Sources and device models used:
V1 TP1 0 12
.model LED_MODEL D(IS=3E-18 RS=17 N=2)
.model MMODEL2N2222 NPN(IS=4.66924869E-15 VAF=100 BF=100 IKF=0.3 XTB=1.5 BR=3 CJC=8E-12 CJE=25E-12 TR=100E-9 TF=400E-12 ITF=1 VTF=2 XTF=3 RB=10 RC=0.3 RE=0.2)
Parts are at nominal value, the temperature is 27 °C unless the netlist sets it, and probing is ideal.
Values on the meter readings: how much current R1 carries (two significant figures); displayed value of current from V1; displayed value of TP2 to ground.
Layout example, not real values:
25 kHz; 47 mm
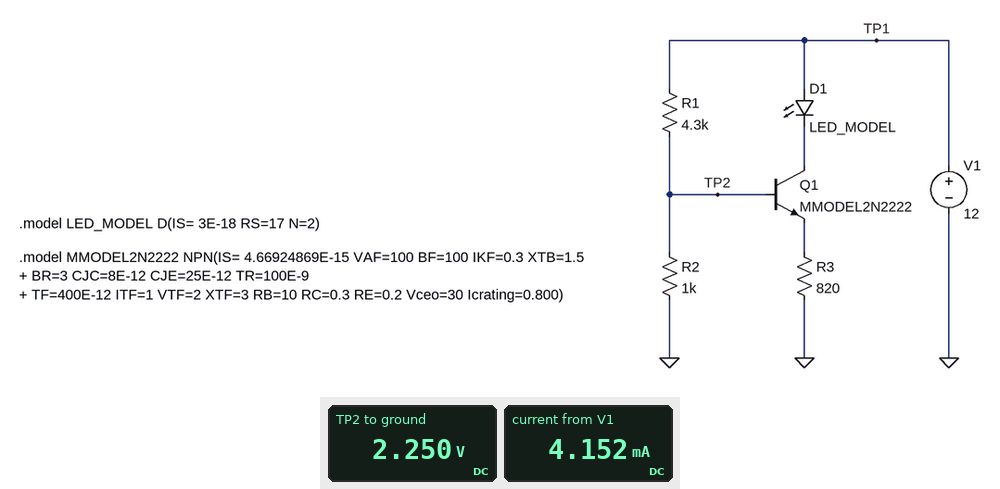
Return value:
2.3 mA; 4.152 mA; 2.250 V
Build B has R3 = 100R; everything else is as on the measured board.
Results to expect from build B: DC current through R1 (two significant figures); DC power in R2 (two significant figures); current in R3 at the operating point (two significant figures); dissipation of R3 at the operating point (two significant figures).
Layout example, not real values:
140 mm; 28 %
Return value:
2.3 mA; 4.6 mW; 14 mA; 20 mW
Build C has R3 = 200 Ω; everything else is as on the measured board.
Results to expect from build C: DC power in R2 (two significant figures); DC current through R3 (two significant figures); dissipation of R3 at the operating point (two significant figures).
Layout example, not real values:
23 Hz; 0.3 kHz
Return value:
4.9 mW; 7.4 mA; 11 mW
